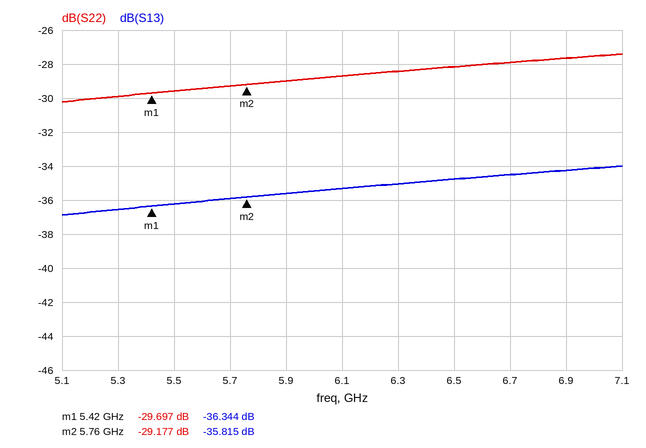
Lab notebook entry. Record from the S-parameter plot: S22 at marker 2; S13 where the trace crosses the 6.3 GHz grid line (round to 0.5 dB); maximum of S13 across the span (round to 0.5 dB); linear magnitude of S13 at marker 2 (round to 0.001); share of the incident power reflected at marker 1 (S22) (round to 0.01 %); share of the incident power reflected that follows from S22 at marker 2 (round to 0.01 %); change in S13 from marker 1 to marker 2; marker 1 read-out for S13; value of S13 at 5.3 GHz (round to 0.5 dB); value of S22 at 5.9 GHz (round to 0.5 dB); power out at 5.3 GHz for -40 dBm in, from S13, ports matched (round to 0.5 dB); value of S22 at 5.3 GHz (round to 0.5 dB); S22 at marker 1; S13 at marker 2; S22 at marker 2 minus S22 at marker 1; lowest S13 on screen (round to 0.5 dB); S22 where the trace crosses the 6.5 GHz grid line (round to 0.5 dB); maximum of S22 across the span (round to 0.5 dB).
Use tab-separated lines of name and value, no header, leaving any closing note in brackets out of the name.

S22 at marker 2	-29.177 dB
S13 where the trace crosses the 6.3 GHz grid line	-35.0 dB
maximum of S13 across the span	-34.0 dB
linear magnitude of S13 at marker 2	0.016
share of the incident power reflected at marker 1 (S22)	0.11 %
share of the incident power reflected that follows from S22 at marker 2	0.12 %
change in S13 from marker 1 to marker 2	0.529 dB
marker 1 read-out for S13	-36.344 dB
value of S13 at 5.3 GHz	-36.5 dB
value of S22 at 5.9 GHz	-29.0 dB
power out at 5.3 GHz for -40 dBm in, from S13, ports matched	-76.5 dBm
value of S22 at 5.3 GHz	-30.0 dB
S22 at marker 1	-29.697 dB
S13 at marker 2	-35.815 dB
S22 at marker 2 minus S22 at marker 1	0.520 dB
lowest S13 on screen	-37.0 dB
S22 where the trace crosses the 6.5 GHz grid line	-28.0 dB
maximum of S22 across the span	-27.5 dB
